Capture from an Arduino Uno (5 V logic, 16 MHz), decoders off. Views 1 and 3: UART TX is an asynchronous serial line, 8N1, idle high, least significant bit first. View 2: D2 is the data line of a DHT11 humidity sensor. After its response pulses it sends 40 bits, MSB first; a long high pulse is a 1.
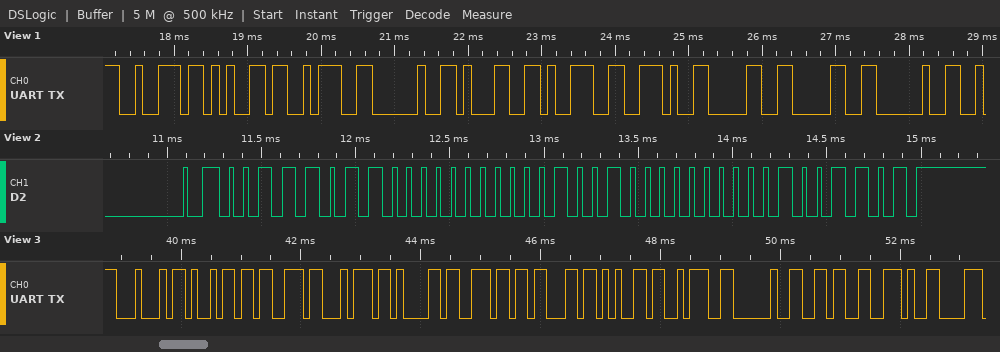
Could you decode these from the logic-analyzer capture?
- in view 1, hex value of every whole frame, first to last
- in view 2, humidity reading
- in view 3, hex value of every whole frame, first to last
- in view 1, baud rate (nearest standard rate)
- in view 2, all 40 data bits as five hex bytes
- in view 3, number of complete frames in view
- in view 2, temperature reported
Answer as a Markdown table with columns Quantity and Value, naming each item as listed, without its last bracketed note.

| Quantity | Value |
|---|---|
| in view 1, hex value of every whole frame, first to last | 72 65 3A 20 31 39 2E 30 30 20 |
| in view 2, humidity reading | 59 % |
| in view 3, hex value of every whole frame, first to last | 44 69 73 74 61 6E 63 65 3A 20 36 2E |
| in view 1, baud rate | 9600 baud |
| in view 2, all 40 data bits as five hex bytes | 3B 00 12 00 4D |
| in view 3, number of complete frames in view | 12 |
| in view 2, temperature reported | 18.0 °C |
